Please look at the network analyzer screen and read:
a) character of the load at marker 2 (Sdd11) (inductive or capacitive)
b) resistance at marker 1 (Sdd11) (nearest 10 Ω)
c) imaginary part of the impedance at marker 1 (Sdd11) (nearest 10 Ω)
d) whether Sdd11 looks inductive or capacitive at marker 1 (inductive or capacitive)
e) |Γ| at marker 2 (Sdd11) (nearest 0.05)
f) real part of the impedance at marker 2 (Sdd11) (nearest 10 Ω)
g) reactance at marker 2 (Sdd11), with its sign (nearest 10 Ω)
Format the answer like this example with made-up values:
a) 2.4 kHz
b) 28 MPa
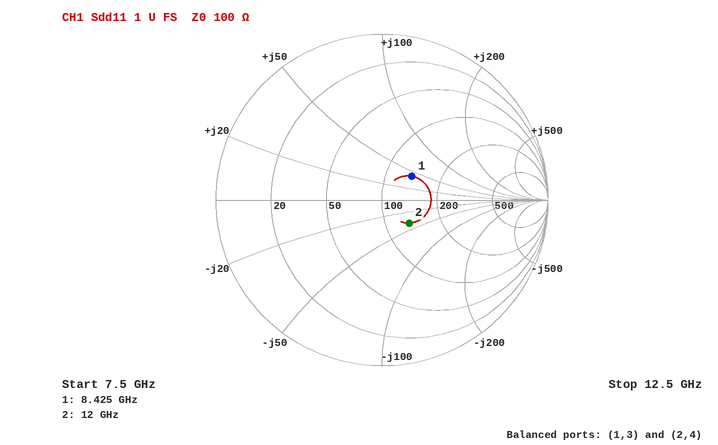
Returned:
a) capacitive
b) 140 Ω
c) +40 Ω
d) inductive
e) 0.20
f) 130 Ω
g) -40 Ω
